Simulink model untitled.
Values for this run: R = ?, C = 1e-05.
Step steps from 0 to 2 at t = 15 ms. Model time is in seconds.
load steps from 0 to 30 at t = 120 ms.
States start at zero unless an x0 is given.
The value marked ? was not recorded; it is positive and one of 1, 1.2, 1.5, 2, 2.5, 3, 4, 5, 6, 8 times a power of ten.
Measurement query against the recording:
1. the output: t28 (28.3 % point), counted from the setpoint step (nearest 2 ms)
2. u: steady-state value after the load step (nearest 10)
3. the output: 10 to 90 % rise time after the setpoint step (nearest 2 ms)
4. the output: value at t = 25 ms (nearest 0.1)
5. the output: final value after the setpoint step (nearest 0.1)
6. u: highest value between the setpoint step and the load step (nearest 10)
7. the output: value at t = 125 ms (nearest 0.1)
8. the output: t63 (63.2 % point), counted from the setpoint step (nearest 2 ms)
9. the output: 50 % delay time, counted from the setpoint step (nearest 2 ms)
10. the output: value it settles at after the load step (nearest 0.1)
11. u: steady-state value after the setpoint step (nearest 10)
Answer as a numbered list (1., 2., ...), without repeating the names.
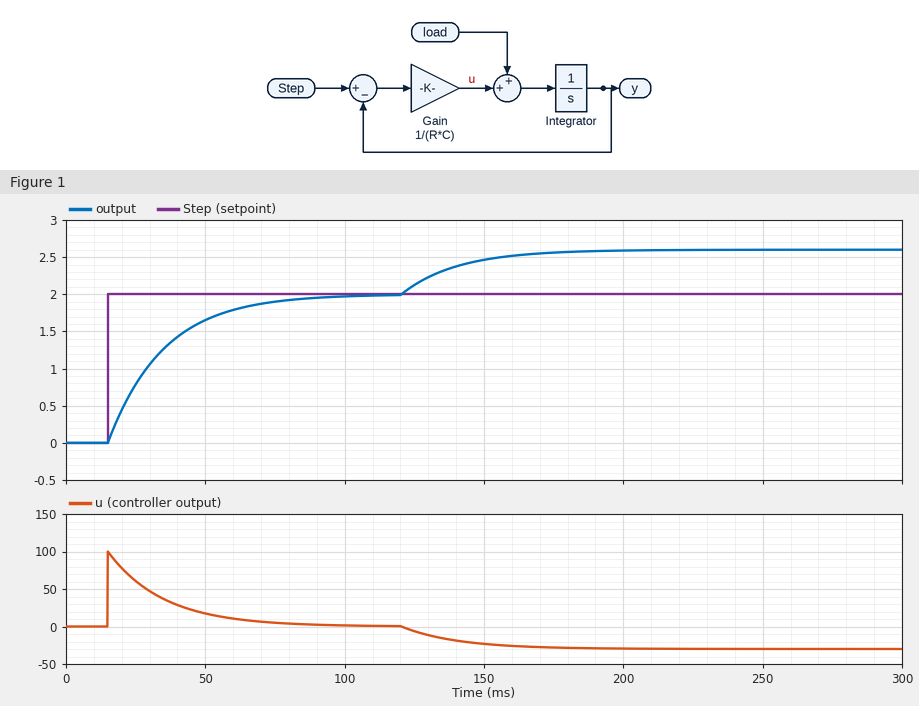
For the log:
1. 6 ms
2. -30
3. 44 ms
4. 0.8
5. 2.0
6. 100
7. 2.1
8. 20 ms
9. 14 ms
10. 2.6
11. 0
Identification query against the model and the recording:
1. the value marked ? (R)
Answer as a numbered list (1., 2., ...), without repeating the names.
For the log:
1. 2000
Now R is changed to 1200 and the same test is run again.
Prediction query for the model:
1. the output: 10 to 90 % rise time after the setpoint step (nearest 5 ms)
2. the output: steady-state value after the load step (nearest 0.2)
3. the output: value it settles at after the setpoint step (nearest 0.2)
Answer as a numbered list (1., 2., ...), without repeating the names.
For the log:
1. 25 ms
2. 2.4
3. 2.0
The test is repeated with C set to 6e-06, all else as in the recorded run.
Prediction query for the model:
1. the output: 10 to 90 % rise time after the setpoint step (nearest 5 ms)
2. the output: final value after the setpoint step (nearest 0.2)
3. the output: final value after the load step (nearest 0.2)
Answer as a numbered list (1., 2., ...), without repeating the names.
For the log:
1. 25 ms
2. 2.0
3. 2.4
